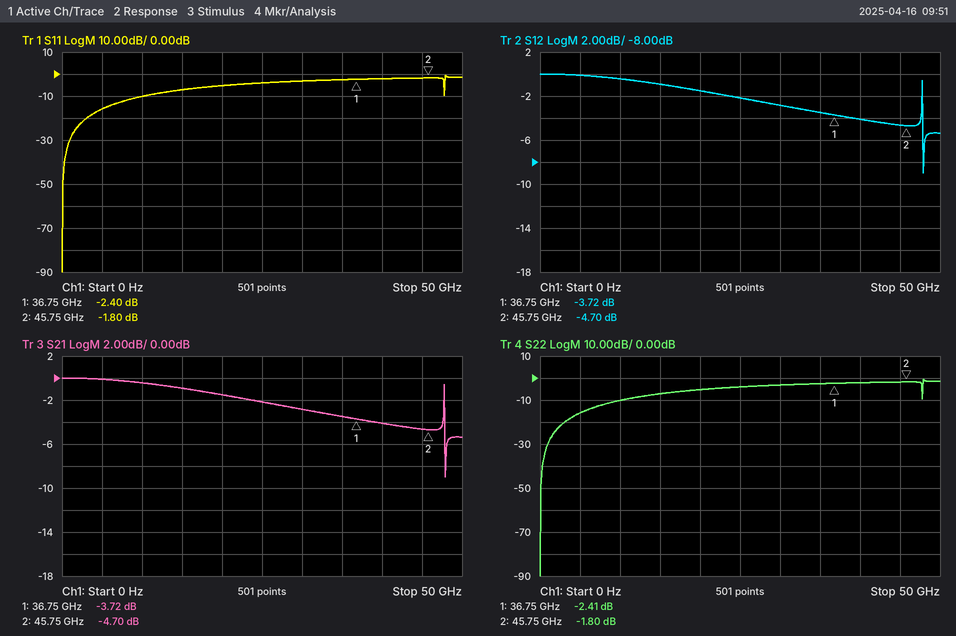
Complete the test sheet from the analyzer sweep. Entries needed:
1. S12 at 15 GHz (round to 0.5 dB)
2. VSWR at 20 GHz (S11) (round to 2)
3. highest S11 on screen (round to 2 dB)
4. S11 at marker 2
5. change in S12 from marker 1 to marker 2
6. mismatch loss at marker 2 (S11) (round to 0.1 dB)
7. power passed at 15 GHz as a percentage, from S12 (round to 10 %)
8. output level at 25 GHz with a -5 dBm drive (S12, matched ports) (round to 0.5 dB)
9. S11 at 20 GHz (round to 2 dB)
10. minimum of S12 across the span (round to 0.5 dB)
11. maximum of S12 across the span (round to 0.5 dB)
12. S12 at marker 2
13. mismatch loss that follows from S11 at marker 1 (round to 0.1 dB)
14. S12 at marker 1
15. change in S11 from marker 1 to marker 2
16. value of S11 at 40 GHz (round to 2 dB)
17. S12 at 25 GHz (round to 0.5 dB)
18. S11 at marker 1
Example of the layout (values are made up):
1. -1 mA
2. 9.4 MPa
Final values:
1. -1.0 dB
2. 4
3. 0 dB
4. -1.80 dB
5. -0.98 dB
6. 4.7 dB
7. 80 %
8. -7.0 dBm
9. -6 dB
10. -9.0 dB
11. 0.0 dB
12. -4.70 dB
13. 3.7 dB
14. -3.72 dB
15. 0.60 dB
16. -2 dB
17. -2.0 dB
18. -2.40 dB
